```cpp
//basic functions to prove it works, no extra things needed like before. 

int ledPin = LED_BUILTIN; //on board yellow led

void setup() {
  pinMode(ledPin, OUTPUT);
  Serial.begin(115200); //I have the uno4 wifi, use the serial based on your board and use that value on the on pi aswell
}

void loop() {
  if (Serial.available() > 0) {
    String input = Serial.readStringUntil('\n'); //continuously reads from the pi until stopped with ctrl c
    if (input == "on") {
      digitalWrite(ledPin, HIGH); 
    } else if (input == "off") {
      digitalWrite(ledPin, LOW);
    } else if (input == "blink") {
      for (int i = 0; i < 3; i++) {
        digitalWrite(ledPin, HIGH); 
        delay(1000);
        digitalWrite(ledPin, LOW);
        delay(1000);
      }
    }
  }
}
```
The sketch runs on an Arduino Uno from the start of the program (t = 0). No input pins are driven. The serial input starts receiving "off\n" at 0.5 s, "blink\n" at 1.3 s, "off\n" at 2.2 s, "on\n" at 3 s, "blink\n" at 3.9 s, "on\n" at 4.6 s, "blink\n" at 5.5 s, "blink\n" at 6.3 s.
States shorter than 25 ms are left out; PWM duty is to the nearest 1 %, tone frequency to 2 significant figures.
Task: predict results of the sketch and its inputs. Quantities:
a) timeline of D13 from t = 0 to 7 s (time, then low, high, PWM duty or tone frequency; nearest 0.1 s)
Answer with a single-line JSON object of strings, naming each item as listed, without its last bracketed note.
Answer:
{"timeline of D13 from t = 0 to 7 s": "0 s low; 1.3 s high; 2.3 s low; 3.3 s high; 4.3 s low; 5.3 s high; 6.3 s low"}
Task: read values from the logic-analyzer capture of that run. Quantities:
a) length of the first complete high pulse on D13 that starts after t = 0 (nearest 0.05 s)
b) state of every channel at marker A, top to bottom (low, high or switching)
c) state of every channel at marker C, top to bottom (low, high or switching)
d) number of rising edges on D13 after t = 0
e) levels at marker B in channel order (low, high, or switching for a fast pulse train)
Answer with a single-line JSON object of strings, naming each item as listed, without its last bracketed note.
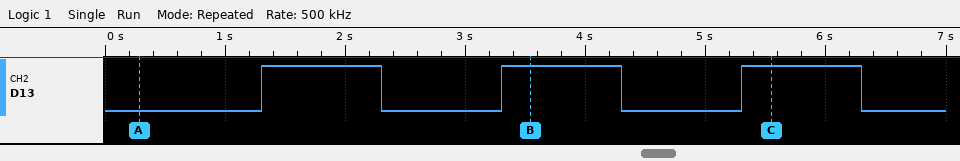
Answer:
{"length of the first complete high pulse on D13 that starts after t = 0": "1.00 s", "state of every channel at marker A, top to bottom": "D13 low", "state of every channel at marker C, top to bottom": "D13 high", "number of rising edges on D13 after t = 0": "3", "levels at marker B in channel order": "D13 high"}
